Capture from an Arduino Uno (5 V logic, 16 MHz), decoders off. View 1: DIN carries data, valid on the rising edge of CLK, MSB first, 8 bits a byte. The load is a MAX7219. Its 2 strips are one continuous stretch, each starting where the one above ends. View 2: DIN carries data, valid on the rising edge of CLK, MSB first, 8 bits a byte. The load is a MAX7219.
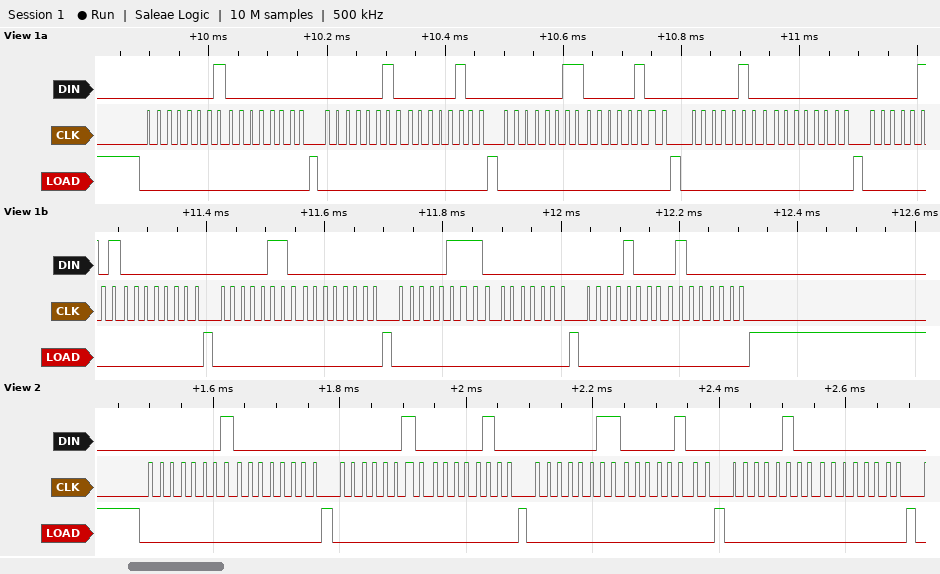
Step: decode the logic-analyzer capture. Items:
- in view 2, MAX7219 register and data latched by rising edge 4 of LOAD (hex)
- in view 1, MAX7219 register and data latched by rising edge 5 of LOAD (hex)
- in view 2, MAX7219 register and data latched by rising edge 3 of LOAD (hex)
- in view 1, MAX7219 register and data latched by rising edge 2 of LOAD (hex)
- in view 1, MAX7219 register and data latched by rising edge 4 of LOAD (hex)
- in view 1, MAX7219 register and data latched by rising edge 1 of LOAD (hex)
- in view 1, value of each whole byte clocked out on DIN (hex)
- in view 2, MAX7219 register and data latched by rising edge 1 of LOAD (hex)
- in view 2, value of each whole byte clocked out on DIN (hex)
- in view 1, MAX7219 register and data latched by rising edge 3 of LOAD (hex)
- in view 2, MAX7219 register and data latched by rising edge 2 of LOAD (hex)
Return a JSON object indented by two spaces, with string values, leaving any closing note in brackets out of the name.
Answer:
{
  "in view 2, MAX7219 register and data latched by rising edge 4 of LOAD": "register 0x4, data 0x00",
  "in view 1, MAX7219 register and data latched by rising edge 5 of LOAD": "register 0x5, data 0x00",
  "in view 2, MAX7219 register and data latched by rising edge 3 of LOAD": "register 0x3, data 0x04",
  "in view 1, MAX7219 register and data latched by rising edge 2 of LOAD": "register 0x2, data 0x04",
  "in view 1, MAX7219 register and data latched by rising edge 4 of LOAD": "register 0x4, data 0x00",
  "in view 1, MAX7219 register and data latched by rising edge 1 of LOAD": "register 0x1, data 0x00",
  "in view 1, value of each whole byte clocked out on DIN": "01 00 02 04 03 04 04 00 05 00 06 00 07 00 08 40",
  "in view 2, MAX7219 register and data latched by rising edge 1 of LOAD": "register 0x1, data 0x00",
  "in view 2, value of each whole byte clocked out on DIN": "0x01 0x00 0x02 0x04 0x03 0x04 0x04 0x00",
  "in view 1, MAX7219 register and data latched by rising edge 3 of LOAD": "register 0x3, data 0x04",
  "in view 2, MAX7219 register and data latched by rising edge 2 of LOAD": "register 0x2, data 0x04"
}
